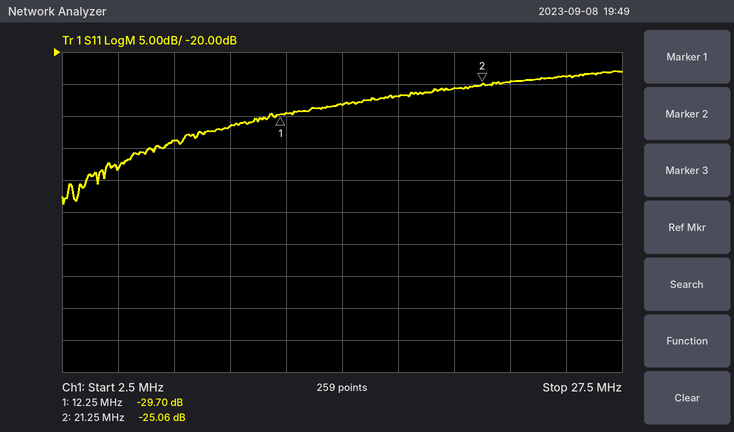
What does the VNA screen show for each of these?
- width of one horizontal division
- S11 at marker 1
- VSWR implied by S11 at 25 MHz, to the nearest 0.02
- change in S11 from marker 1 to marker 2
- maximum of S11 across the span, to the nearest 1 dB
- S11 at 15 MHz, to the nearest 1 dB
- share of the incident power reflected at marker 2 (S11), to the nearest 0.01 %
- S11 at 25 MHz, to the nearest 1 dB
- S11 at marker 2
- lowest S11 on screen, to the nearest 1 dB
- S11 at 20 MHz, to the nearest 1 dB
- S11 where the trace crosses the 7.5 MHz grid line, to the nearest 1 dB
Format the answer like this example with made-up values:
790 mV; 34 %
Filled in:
2.5 MHz; -29.70 dB; 1.14; 4.64 dB; -23 dB; -28 dB; 0.31 %; -24 dB; -25.06 dB; -44 dB; -26 dB; -34 dB
